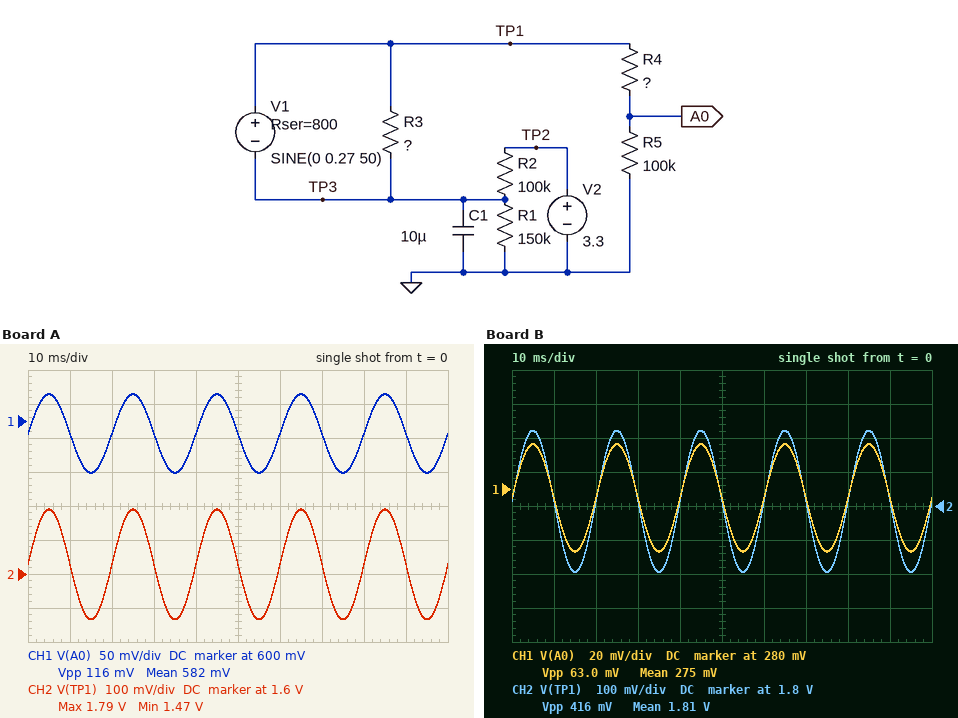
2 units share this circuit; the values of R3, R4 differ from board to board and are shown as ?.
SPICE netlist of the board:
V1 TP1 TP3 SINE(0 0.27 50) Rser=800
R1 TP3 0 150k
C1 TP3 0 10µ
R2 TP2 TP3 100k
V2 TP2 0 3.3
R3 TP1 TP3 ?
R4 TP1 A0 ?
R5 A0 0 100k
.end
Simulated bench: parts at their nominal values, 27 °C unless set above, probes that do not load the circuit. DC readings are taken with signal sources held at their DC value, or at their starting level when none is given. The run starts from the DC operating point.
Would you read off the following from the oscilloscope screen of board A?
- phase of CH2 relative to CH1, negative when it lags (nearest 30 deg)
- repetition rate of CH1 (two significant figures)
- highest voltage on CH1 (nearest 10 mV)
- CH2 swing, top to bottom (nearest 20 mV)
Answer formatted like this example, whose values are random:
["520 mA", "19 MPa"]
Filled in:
["0 deg", "50 Hz", "640 mV", "320 mV"]
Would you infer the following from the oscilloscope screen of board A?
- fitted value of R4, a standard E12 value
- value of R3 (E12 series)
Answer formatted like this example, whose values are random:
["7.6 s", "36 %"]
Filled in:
["180 kΩ", "1.2 kΩ"]
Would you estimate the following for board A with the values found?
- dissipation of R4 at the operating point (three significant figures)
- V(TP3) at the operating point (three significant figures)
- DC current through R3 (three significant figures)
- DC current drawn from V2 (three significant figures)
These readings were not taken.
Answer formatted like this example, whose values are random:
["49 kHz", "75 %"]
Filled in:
["6.09 µW", "1.63 V", "2.33 µA", "16.7 µA"]
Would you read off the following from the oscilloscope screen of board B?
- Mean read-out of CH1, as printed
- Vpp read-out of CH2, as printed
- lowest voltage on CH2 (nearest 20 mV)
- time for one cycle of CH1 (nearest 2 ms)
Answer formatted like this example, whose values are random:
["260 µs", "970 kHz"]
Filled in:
["275 mV", "416 mV", "1.60 V", "20 ms"]
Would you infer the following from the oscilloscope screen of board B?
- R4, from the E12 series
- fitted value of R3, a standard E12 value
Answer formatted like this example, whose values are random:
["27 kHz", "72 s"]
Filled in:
["560 kΩ", "2.7 kΩ"]
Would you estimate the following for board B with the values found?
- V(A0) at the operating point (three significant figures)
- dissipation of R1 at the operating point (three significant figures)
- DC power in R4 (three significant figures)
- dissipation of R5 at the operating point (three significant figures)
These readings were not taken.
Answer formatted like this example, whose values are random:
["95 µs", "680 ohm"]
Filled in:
["275 mV", "22.0 µW", "4.23 µW", "755 nW"]
